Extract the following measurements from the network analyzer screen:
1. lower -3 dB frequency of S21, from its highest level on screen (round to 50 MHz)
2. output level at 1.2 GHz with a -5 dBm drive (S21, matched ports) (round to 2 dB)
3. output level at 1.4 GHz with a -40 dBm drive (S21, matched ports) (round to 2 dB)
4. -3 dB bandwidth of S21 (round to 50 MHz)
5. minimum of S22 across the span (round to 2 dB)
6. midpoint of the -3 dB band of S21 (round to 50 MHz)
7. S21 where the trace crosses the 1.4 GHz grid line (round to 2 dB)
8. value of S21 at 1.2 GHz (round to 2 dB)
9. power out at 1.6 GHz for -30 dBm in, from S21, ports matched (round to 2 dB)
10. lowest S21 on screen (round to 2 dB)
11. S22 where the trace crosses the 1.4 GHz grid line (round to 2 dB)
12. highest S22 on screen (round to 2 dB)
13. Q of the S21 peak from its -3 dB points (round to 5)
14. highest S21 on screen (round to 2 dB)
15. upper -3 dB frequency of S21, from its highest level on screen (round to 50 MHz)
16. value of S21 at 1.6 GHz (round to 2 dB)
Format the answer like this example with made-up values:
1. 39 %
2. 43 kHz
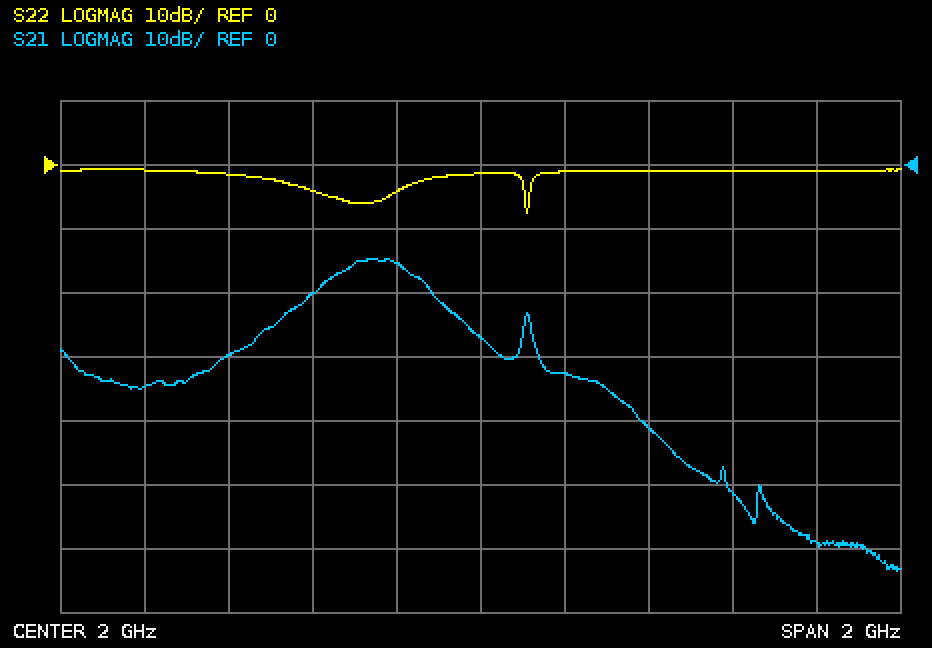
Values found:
1. 1.65 GHz
2. -40 dBm
3. -70 dBm
4. 200 MHz
5. -8 dB
6. 1.75 GHz
7. -30 dB
8. -34 dB
9. -50 dBm
10. -64 dB
11. -2 dB
12. 0 dB
13. 10
14. -14 dB
15. 1.85 GHz
16. -20 dB
